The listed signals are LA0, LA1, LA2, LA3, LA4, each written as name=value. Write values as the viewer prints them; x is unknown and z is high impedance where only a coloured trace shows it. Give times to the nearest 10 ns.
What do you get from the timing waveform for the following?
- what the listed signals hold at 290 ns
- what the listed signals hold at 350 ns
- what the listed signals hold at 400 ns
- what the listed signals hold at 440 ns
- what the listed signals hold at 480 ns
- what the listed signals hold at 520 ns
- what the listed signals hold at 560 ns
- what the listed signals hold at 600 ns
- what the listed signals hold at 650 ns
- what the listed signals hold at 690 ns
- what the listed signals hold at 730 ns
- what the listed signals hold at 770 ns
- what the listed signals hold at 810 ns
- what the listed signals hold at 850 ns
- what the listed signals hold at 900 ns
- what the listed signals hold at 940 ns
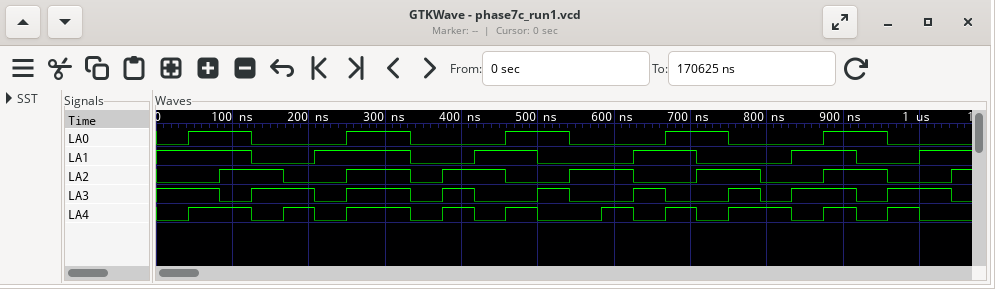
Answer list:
LA0=1, LA1=1, LA2=1, LA3=1, LA4=1
LA0=0, LA1=0, LA2=0, LA3=0, LA4=0
LA0=0, LA1=0, LA2=1, LA3=1, LA4=1
LA0=0, LA1=1, LA2=1, LA3=0, LA4=0
LA0=1, LA1=1, LA2=0, LA3=0, LA4=1
LA0=1, LA1=0, LA2=0, LA3=1, LA4=0
LA0=0, LA1=0, LA2=1, LA3=0, LA4=0
LA0=0, LA1=0, LA2=1, LA3=0, LA4=1
LA0=0, LA1=1, LA2=0, LA3=1, LA4=0
LA0=1, LA1=1, LA2=0, LA3=0, LA4=1
LA0=1, LA1=0, LA2=1, LA3=0, LA4=0
LA0=0, LA1=0, LA2=1, LA3=1, LA4=1
LA0=0, LA1=0, LA2=0, LA3=0, LA4=1
LA0=0, LA1=1, LA2=0, LA3=1, LA4=0
LA0=1, LA1=1, LA2=1, LA3=1, LA4=1
LA0=1, LA1=0, LA2=1, LA3=0, LA4=0
